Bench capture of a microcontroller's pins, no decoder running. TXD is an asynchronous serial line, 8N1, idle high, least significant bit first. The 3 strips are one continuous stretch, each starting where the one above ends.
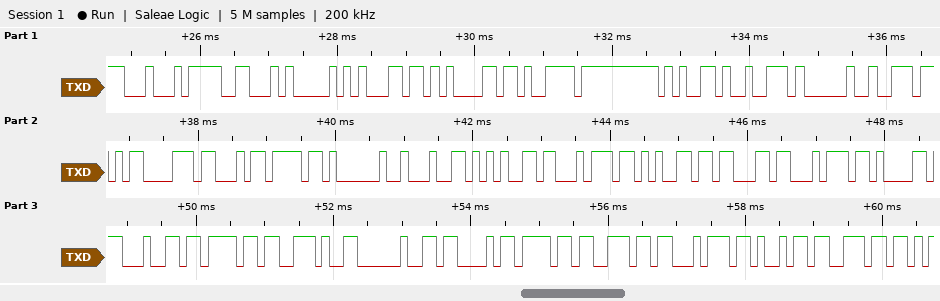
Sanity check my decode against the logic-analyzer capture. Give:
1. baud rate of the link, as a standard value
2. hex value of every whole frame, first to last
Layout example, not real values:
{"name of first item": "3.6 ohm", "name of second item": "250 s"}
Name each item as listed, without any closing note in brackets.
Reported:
{"baud rate of the link, as a standard value": "9600 baud", "hex value of every whole frame, first to last": "0x44 0x46 0x50 0x6C 0x61 0x79 0x65 0x72 0x20 0x6E 0xC3 0xA3 0x6F 0x20 0x64 0x65 0x74 0x65 0x63 0x74 0x61 0x64 0x6F 0x2E 0x20 0x43 0x6F 0x6E 0x74 0x69 0x6E"}
